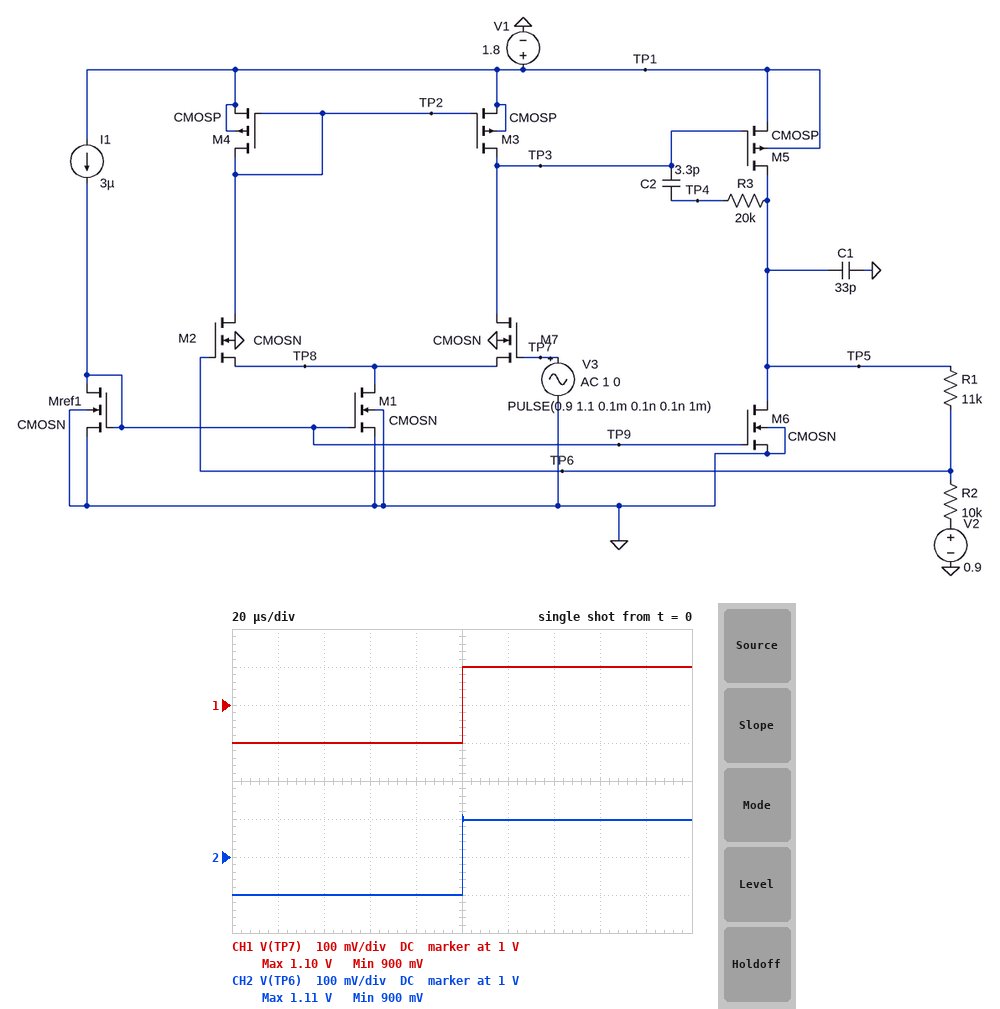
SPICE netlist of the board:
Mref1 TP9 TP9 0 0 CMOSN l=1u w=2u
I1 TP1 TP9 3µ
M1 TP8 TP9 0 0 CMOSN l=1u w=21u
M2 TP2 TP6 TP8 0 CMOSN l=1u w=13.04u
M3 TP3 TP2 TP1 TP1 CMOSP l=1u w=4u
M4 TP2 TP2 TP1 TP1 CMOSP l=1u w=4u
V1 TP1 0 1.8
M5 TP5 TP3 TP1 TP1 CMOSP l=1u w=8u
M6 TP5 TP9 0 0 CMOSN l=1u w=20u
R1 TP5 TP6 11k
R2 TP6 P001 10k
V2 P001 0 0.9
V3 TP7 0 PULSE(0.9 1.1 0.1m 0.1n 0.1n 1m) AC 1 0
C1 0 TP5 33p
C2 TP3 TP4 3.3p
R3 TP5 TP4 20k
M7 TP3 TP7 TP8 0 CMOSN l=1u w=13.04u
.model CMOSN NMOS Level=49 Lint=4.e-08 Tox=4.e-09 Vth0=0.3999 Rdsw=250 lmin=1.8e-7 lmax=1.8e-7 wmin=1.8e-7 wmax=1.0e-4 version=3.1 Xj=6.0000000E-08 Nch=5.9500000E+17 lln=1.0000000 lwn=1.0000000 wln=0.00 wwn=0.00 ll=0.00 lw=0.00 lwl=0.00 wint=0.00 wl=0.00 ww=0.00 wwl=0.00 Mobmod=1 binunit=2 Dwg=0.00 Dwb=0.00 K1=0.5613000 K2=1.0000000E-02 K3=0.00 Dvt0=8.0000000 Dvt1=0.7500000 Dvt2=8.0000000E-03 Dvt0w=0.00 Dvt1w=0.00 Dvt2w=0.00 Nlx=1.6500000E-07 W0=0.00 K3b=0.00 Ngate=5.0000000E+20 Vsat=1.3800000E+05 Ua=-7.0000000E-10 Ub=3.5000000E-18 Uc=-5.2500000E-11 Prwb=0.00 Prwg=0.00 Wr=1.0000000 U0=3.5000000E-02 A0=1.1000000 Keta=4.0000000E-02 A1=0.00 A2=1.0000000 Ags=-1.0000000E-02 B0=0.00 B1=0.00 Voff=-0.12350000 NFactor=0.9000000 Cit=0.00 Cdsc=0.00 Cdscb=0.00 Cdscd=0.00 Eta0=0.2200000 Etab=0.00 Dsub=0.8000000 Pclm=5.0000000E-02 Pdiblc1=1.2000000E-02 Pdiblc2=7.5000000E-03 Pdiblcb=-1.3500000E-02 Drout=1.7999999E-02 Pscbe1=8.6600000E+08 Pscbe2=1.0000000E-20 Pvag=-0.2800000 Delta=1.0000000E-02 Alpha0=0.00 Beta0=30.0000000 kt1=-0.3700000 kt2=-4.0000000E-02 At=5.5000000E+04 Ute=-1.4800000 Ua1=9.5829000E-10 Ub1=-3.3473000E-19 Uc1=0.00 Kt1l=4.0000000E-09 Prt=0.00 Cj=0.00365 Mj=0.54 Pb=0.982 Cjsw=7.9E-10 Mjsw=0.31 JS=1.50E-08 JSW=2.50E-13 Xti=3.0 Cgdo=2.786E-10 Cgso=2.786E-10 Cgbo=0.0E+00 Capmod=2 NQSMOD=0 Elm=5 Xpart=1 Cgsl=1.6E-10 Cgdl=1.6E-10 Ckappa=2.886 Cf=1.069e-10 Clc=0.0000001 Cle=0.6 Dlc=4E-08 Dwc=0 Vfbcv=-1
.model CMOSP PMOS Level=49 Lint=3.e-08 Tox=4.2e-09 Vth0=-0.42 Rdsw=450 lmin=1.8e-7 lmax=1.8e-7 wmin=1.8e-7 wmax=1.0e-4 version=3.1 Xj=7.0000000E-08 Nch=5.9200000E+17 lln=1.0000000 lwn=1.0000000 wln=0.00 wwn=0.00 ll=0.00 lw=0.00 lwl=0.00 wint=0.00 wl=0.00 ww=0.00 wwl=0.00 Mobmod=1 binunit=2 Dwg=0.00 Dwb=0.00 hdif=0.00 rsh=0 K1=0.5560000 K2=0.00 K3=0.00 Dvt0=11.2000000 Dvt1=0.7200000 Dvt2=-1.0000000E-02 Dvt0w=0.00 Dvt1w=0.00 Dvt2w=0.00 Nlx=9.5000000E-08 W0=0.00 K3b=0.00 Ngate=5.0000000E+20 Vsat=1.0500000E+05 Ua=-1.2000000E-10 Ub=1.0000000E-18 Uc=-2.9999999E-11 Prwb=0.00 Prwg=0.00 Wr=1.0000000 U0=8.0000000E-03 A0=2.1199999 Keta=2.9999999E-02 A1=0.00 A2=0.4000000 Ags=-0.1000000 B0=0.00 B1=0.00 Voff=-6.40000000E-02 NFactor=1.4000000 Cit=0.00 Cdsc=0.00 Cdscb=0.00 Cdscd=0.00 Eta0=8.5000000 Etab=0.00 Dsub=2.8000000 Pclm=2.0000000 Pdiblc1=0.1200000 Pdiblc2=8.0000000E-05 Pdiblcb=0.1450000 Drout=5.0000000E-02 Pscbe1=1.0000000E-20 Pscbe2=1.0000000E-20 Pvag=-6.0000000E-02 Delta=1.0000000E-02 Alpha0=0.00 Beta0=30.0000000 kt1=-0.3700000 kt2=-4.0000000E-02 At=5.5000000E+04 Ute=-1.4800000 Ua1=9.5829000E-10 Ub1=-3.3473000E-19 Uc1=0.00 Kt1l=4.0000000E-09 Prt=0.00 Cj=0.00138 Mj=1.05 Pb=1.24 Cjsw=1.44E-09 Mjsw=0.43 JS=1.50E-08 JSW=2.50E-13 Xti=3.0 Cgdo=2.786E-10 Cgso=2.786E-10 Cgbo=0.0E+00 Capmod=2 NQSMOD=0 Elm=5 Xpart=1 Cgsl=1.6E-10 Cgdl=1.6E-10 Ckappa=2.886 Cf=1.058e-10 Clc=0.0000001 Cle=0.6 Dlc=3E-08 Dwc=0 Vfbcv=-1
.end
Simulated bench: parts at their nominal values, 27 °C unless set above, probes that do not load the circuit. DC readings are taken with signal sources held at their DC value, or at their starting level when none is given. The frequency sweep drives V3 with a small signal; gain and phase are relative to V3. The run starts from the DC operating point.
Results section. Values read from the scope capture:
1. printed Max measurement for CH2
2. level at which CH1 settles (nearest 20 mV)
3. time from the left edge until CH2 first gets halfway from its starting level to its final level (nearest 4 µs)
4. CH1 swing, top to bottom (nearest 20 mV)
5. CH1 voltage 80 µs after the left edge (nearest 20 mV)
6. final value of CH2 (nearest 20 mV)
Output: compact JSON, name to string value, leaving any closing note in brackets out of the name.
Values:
{"printed Max measurement for CH2": "1.11 V", "level at which CH1 settles": "1.10 V", "time from the left edge until CH2 first gets halfway from its starting level to its final level": "100 µs", "CH1 swing, top to bottom": "200 mV", "CH1 voltage 80 µs after the left edge": "900 mV", "final value of CH2": "1.10 V"}
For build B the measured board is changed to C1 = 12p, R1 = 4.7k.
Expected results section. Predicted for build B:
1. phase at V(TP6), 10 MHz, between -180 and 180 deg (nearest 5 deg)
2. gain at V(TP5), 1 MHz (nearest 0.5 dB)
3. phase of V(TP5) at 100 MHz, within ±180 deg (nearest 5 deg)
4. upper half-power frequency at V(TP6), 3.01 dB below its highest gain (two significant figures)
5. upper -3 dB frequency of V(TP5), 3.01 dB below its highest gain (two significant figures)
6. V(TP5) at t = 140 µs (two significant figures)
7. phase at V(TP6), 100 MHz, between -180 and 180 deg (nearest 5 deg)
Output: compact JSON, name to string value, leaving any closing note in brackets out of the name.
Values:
{"phase at V(TP6), 10 MHz, between -180 and 180 deg": "-80 deg", "gain at V(TP5), 1 MHz": "3.0 dB", "phase of V(TP5) at 100 MHz, within ±180 deg": "-155 deg", "upper half-power frequency at V(TP6), 3.01 dB below its highest gain": "4.6 MHz", "upper -3 dB frequency of V(TP5), 3.01 dB below its highest gain": "4.7 MHz", "V(TP5) at t = 140 µs": "1.2 V", "phase at V(TP6), 100 MHz, between -180 and 180 deg": "90 deg"}
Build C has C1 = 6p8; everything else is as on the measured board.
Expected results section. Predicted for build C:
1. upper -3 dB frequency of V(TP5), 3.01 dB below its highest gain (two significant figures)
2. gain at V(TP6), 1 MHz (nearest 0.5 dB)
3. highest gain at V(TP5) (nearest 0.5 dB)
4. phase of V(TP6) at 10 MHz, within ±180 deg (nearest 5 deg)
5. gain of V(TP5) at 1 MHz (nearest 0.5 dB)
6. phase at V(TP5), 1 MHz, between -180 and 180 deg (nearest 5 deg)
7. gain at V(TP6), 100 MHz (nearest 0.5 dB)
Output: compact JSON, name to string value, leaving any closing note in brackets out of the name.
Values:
{"upper -3 dB frequency of V(TP5), 3.01 dB below its highest gain": "3.8 MHz", "gain at V(TP6), 1 MHz": "-0.5 dB", "highest gain at V(TP5)": "6.5 dB", "phase of V(TP6) at 10 MHz, within ±180 deg": "-70 deg", "gain of V(TP5) at 1 MHz": "6.0 dB", "phase at V(TP5), 1 MHz, between -180 and 180 deg": "-15 deg", "gain at V(TP6), 100 MHz": "-20.0 dB"}
